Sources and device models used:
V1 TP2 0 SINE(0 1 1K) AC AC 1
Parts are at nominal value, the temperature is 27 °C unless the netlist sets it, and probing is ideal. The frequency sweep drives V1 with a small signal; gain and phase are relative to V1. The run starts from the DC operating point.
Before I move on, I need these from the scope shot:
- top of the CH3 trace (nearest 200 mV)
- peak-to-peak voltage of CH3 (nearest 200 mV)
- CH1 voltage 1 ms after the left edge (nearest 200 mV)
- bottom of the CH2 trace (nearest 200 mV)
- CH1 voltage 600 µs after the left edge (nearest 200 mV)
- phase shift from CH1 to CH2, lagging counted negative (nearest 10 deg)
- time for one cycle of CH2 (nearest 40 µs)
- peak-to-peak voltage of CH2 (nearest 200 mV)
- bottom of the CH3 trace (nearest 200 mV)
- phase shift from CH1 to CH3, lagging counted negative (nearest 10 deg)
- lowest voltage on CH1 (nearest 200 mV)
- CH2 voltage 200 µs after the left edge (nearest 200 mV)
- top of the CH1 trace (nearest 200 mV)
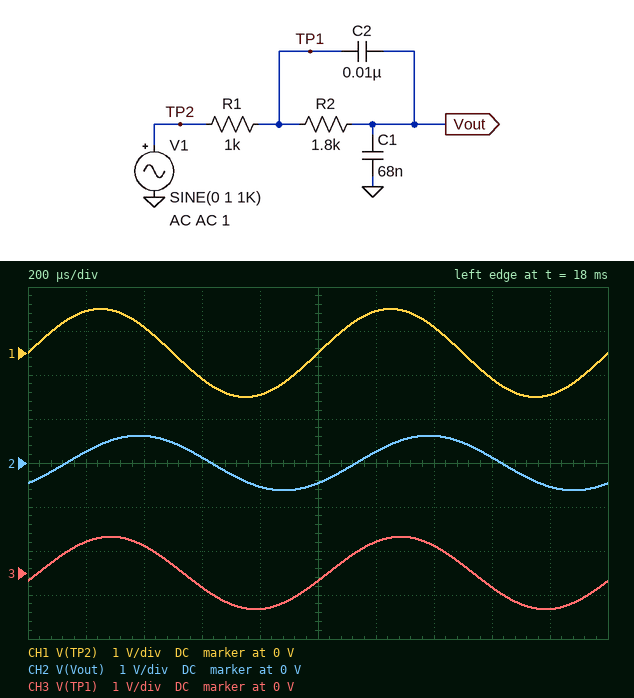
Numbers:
800 mV
1.6 V
0 V
-600 mV
-600 mV
-50 deg
1.00 ms
1.2 V
-800 mV
-10 deg
-1.0 V
200 mV
1.0 V
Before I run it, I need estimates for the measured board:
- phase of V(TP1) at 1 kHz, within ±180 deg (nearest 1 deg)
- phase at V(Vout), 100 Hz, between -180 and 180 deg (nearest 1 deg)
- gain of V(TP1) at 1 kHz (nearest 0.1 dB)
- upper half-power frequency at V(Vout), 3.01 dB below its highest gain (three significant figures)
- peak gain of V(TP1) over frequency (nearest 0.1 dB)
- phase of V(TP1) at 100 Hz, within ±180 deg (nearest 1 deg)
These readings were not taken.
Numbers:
-13 deg
-7 deg
-1.7 dB
792 Hz
0 dB
-2 deg
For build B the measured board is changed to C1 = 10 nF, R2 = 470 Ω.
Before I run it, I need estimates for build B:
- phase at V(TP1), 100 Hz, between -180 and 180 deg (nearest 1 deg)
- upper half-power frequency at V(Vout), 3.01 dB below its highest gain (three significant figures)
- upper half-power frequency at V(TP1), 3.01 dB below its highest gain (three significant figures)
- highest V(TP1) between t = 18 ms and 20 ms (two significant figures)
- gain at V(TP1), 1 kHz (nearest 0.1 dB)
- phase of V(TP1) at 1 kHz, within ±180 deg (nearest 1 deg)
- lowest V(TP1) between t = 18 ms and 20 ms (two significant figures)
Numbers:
0 deg
10.1 kHz
14.3 kHz
1.0 V
0 dB
-4 deg
-1.0 V
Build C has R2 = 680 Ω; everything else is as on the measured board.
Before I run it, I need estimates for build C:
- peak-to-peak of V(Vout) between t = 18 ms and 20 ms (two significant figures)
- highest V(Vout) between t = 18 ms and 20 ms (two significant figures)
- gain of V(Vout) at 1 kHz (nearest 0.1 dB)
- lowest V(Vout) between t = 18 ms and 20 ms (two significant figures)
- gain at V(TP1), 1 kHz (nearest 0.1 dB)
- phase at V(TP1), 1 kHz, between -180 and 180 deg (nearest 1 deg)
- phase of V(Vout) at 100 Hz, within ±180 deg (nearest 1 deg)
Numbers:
1.6 V
810 mV
-1.9 dB
-810 mV
-1.4 dB
-19 deg
-4 deg
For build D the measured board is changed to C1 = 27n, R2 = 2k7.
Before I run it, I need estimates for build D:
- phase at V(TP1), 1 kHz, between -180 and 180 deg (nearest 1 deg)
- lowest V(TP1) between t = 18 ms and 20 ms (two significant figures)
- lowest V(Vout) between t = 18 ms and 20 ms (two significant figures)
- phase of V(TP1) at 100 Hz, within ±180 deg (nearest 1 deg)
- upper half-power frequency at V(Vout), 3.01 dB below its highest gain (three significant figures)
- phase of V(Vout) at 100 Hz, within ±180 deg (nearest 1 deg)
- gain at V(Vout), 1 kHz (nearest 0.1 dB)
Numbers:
-7 deg
-940 mV
-810 mV
-1 deg
1.38 kHz
-4 deg
-1.9 dB
